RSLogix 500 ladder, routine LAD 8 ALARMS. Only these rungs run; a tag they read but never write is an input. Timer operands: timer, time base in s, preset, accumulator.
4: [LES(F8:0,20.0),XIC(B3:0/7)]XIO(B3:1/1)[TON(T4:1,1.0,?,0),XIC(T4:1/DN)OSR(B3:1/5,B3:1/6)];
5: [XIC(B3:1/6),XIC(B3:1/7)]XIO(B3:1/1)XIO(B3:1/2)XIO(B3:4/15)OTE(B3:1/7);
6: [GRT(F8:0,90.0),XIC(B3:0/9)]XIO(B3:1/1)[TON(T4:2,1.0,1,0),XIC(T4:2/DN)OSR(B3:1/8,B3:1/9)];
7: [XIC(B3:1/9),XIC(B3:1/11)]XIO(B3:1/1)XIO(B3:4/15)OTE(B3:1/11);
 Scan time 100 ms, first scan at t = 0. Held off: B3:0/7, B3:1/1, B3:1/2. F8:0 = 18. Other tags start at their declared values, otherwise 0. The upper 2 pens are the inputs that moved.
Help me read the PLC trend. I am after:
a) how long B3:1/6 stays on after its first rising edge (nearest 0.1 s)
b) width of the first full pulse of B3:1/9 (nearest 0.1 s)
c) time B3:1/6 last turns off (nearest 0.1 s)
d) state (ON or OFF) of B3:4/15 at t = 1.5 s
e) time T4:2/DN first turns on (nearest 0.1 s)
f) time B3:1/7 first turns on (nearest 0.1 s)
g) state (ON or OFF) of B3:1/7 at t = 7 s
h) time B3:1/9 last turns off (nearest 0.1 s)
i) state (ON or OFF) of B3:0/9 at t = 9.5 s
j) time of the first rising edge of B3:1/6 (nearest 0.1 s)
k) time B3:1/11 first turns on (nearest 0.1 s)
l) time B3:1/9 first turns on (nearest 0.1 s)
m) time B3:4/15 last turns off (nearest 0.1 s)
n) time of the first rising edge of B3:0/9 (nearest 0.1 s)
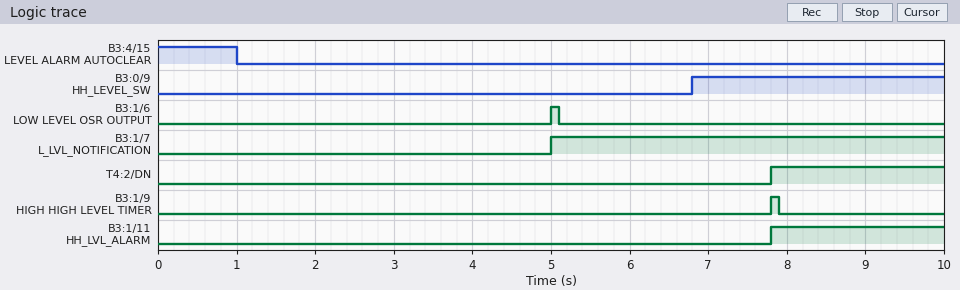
0.1 s
0.1 s
5.1 s
OFF
7.8 s
5.0 s
ON
7.9 s
ON
5.0 s
7.8 s
7.8 s
1.0 s
6.8 s
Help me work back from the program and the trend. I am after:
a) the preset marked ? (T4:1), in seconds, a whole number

5 s
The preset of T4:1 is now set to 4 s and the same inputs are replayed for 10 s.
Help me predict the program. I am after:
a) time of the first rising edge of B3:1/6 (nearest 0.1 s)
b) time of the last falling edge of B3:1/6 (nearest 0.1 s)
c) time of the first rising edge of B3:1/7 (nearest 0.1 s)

4.0 s
4.1 s
4.0 s
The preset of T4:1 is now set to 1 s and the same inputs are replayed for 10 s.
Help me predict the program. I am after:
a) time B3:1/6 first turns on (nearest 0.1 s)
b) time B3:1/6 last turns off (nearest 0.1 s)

1.0 s
1.1 s
